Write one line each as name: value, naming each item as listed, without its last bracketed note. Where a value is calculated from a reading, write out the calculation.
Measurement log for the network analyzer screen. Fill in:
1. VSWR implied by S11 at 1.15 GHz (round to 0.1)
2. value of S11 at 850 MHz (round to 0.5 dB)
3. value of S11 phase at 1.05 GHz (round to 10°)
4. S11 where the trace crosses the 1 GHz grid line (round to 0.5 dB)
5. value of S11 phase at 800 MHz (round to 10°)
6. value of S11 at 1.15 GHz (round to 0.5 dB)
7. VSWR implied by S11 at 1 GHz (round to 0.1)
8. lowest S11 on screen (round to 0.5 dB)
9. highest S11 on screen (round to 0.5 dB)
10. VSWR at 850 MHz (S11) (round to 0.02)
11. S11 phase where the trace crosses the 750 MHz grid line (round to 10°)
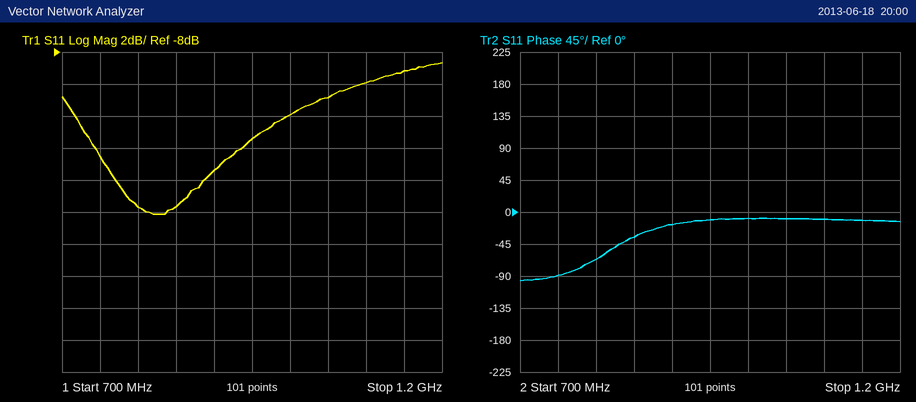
VSWR implied by S11 at 1.15 GHz: |Γ| = 10^(-9/20) = 0.3548; VSWR = (1 + 0.3548)/(1 − 0.3548) ≈ 2.1
value of S11 at 850 MHz: -17.5 dB
value of S11 phase at 1.05 GHz: -10°
S11 where the trace crosses the 1 GHz grid line: -12.0 dB
value of S11 phase at 800 MHz: -70°
value of S11 at 1.15 GHz: -9.0 dB
VSWR implied by S11 at 1 GHz: |Γ| = 10^(-12/20) = 0.2512; VSWR = (1 + 0.2512)/(1 − 0.2512) ≈ 1.7
lowest S11 on screen: -18.0 dB
highest S11 on screen: -8.5 dB
VSWR at 850 MHz (S11): |Γ| = 10^(-17.5/20) = 0.1334; VSWR = (1 + 0.1334)/(1 − 0.1334) ≈ 1.31, so 1.30 to the nearest 0.02
S11 phase where the trace crosses the 750 MHz grid line: -90°
